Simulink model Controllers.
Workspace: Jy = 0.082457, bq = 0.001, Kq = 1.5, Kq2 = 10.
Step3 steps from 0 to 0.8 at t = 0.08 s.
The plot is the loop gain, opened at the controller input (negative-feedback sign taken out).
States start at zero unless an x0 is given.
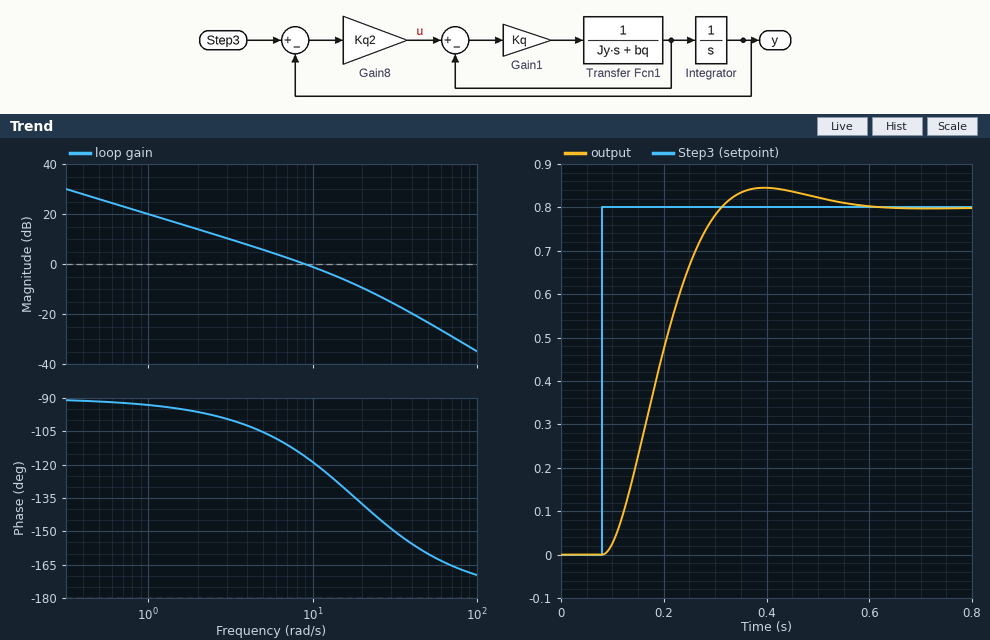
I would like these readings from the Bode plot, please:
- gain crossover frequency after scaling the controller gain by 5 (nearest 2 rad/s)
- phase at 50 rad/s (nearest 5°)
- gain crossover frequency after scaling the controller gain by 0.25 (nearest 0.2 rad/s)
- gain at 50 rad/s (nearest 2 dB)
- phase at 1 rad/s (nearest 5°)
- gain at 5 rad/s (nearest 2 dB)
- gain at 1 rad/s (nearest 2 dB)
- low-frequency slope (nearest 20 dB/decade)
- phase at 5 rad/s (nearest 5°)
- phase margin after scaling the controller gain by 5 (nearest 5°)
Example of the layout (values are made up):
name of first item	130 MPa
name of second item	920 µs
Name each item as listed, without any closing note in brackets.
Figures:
gain crossover frequency after scaling the controller gain by 5	28 rad/s
phase at 50 rad/s	-160°
gain crossover frequency after scaling the controller gain by 0.25	2.4 rad/s
gain at 50 rad/s	-24 dB
phase at 1 rad/s	-95°
gain at 5 rad/s	6 dB
gain at 1 rad/s	20 dB
low-frequency slope	-20 dB/decade
phase at 5 rad/s	-105°
phase margin after scaling the controller gain by 5	35°
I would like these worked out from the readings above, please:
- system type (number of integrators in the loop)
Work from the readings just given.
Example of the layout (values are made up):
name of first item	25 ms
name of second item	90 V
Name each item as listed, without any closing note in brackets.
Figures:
system type	1
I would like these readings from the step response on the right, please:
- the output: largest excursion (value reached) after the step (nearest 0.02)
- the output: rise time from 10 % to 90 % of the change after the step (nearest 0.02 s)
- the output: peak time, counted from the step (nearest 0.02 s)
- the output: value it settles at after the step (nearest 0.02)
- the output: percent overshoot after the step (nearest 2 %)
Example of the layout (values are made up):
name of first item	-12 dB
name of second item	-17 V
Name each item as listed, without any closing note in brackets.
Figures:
the output: largest excursion (value reached) after the step	0.84
the output: rise time from 10 % to 90 % of the change after the step	0.16 s
the output: peak time, counted from the step	0.32 s
the output: value it settles at after the step	0.80
the output: percent overshoot after the step	6 %
